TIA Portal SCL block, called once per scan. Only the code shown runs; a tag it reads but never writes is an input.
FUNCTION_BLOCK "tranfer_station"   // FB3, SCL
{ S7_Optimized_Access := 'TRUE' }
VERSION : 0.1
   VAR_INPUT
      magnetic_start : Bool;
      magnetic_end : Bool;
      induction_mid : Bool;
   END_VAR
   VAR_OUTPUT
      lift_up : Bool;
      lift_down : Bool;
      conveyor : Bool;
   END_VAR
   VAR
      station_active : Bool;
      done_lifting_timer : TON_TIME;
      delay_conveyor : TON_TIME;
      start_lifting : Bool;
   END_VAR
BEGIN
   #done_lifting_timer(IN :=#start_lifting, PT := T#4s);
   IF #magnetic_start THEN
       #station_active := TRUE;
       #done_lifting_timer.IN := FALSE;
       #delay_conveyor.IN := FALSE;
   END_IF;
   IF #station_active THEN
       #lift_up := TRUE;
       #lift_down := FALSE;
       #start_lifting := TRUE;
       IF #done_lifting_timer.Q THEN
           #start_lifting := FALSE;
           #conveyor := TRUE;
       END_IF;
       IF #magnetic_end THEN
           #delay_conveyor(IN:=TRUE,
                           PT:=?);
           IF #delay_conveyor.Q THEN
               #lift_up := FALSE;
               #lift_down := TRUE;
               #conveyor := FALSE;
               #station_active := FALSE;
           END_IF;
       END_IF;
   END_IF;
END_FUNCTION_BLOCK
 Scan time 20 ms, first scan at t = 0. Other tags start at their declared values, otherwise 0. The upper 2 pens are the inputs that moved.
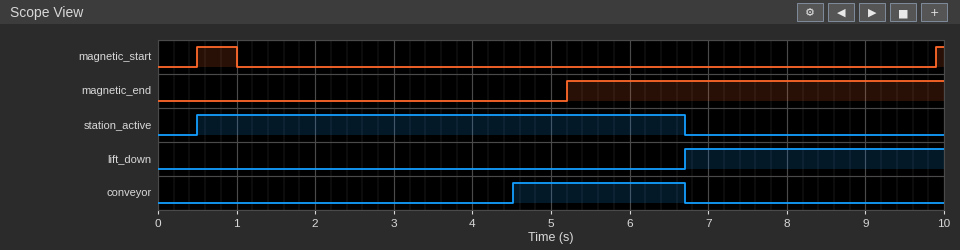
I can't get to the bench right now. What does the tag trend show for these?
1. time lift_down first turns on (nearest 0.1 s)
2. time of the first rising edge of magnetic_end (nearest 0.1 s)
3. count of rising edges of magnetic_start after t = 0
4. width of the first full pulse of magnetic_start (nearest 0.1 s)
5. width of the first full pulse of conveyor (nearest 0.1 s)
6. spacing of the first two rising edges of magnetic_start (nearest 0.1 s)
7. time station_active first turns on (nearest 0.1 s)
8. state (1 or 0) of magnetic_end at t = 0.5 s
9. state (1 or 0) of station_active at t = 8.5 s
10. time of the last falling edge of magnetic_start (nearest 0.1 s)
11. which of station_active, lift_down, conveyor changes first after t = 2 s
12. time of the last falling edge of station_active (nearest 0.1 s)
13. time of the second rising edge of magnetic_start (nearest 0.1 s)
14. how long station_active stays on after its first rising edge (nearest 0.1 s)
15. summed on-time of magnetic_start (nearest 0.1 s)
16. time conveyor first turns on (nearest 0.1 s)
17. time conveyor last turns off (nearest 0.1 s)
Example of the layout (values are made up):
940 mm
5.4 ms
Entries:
6.7 s
5.2 s
2
0.5 s
2.2 s
9.4 s
0.5 s
0
0
1.0 s
conveyor
6.7 s
9.9 s
6.2 s
0.6 s
4.5 s
6.7 s
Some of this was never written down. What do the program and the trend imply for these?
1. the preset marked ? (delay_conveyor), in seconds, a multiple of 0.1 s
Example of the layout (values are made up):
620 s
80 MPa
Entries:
1.5 s
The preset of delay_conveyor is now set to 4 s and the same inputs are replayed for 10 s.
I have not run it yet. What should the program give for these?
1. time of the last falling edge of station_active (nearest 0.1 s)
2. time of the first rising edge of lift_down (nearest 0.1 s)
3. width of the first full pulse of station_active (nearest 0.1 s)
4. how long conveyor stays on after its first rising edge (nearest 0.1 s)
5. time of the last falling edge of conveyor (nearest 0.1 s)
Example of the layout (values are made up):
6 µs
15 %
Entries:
9.2 s
9.2 s
8.7 s
4.7 s
9.2 s
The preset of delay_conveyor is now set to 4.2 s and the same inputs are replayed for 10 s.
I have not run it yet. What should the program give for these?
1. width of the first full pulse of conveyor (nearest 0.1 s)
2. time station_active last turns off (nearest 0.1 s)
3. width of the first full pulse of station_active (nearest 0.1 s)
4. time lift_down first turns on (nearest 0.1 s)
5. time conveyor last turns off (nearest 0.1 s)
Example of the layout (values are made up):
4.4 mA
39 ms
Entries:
4.9 s
9.4 s
8.9 s
9.4 s
9.4 s
